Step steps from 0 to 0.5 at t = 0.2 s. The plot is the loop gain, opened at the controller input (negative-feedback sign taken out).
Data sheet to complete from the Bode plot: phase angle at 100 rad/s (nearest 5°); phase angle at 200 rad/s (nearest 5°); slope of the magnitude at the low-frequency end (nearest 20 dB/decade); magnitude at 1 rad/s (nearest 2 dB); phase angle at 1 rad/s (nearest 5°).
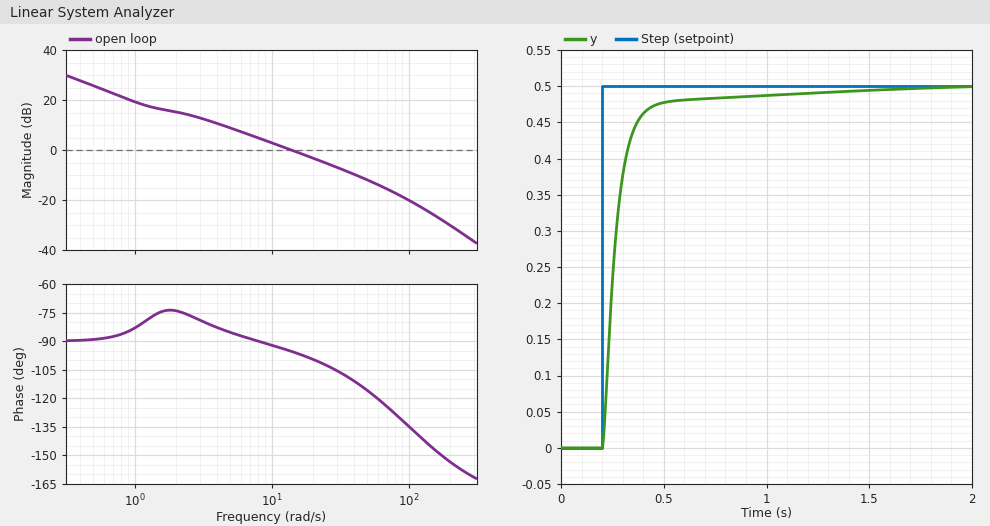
-135°
-155°
-20 dB/decade
20 dB
-85°
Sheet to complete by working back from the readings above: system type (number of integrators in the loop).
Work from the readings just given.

1
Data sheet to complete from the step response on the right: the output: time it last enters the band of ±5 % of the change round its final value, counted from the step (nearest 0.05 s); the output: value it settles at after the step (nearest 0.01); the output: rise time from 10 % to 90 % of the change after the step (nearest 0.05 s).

0.25 s
0.50
0.15 s
